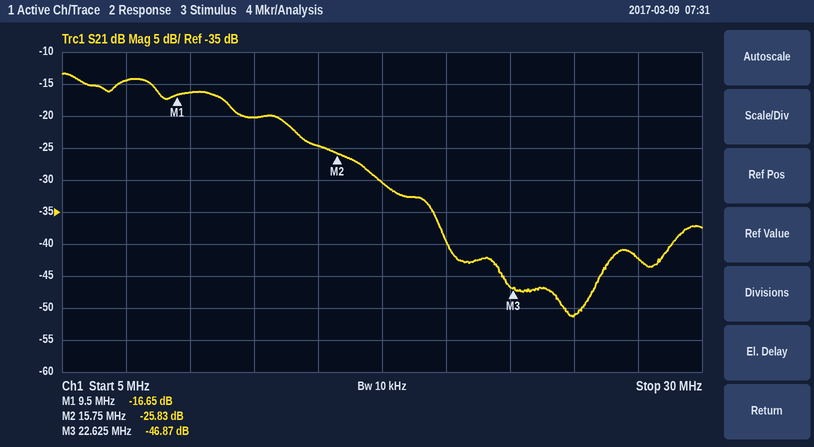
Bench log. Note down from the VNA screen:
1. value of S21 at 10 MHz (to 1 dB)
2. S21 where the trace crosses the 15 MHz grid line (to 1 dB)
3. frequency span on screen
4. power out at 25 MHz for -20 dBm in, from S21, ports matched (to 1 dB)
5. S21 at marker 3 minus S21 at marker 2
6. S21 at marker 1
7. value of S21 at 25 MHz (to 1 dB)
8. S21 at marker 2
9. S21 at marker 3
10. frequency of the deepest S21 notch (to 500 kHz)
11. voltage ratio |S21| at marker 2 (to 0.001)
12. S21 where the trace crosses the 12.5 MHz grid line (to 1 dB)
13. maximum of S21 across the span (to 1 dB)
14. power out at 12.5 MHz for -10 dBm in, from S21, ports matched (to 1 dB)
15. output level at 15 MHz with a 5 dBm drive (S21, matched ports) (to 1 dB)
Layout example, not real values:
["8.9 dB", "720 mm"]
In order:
["-16 dB", "-25 dB", "25 MHz", "-71 dBm", "-21.04 dB", "-16.65 dB", "-51 dB", "-25.83 dB", "-46.87 dB", "25.0 MHz", "0.051", "-20 dB", "-13 dB", "-30 dBm", "-20 dBm"]
